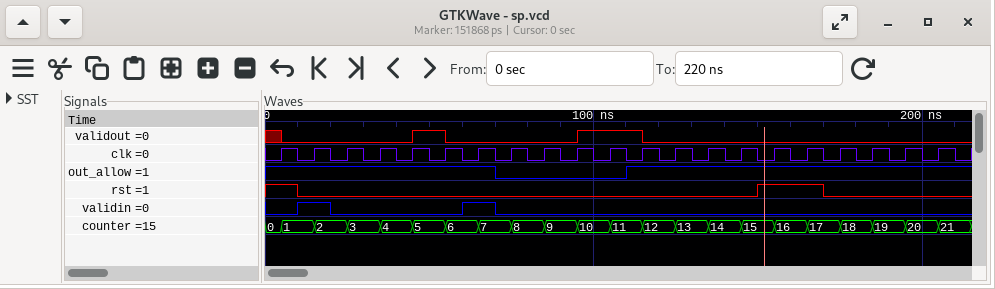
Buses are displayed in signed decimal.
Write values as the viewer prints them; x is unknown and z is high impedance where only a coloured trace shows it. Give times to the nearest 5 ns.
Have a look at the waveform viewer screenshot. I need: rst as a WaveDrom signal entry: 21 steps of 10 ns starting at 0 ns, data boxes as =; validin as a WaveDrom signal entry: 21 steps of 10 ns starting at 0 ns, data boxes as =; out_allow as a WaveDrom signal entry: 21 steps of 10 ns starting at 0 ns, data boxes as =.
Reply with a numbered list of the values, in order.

1. {name: 'rst', wave: '10.............1.0...'}
2. {name: 'validin', wave: '010...10.............'}
3. {name: 'out_allow', wave: '1......0...1.........'}
